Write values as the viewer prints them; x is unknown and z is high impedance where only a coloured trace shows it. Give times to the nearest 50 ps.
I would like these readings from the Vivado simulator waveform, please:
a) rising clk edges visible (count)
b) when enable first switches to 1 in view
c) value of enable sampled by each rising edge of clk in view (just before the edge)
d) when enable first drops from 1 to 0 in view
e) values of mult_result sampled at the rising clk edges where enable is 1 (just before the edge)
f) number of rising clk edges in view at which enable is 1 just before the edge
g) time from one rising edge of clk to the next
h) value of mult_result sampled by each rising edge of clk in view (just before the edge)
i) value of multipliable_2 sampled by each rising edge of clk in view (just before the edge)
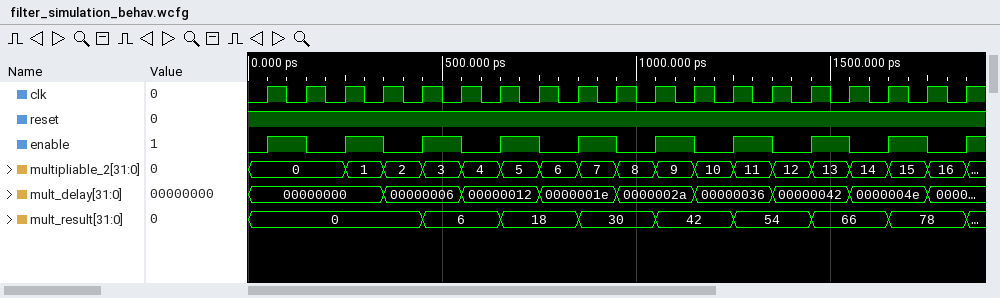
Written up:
19
50 ps
0 1 0 1 0 1 0 1 0 1 0 1 0 1 0 1 0 1 0
150 ps
0, 0, 6, 18, 30, 42, 54, 66, 78
9
100 ps
0, 0, 0, 0, 0, 6, 6, 18, 18, 30, 30, 42, 42, 54, 54, 66, 66, 78, 78
0, 0, 0, 1, 2, 3, 4, 5, 6, 7, 8, 9, 10, 11, 12, 13, 14, 15, 16
